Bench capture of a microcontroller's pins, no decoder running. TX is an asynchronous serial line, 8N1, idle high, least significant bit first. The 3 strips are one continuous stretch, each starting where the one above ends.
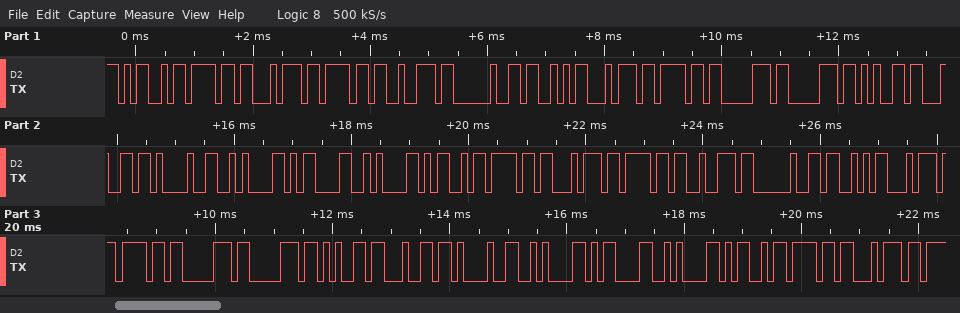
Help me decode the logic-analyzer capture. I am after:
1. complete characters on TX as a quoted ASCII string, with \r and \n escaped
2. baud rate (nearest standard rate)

"Motor Stopped!\n\r\nMotor Stopped!\n\r\nMot"
9600 baud
